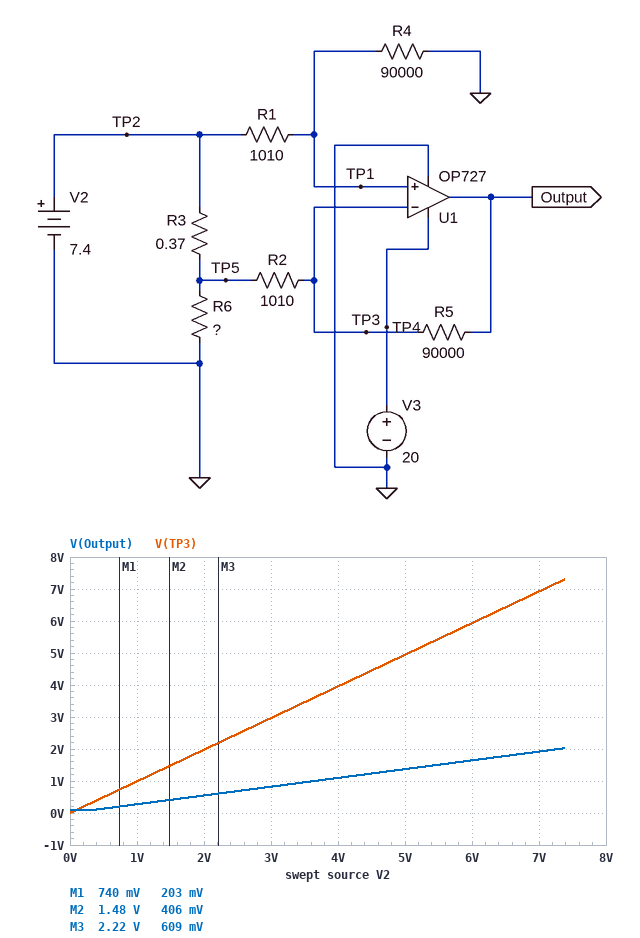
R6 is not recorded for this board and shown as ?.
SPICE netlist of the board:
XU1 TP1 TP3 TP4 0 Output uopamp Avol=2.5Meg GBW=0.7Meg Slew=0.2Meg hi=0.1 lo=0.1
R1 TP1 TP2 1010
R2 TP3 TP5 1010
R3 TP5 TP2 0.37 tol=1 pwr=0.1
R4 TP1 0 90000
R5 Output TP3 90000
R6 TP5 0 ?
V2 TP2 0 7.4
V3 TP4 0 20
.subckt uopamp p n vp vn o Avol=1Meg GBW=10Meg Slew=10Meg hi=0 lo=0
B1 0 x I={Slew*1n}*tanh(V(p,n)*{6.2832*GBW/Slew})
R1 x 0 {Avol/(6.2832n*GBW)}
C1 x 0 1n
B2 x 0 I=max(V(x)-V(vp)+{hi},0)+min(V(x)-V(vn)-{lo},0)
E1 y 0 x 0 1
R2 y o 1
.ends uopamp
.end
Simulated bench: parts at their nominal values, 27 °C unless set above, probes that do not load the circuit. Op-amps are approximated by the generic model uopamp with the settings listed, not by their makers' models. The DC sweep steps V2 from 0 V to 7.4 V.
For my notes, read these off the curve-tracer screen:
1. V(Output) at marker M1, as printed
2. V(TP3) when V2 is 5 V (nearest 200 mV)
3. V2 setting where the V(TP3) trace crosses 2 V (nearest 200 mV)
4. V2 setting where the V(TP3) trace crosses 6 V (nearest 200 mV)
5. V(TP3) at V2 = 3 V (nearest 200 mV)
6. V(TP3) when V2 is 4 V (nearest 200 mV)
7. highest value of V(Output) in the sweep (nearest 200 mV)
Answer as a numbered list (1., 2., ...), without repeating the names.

1. 203 mV
2. 5.0 V
3. 2.0 V
4. 6.0 V
5. 3.0 V
6. 4.0 V
7. 2.0 V
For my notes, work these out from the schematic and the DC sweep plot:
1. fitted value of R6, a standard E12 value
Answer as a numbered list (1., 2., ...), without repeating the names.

1. 120 Ω
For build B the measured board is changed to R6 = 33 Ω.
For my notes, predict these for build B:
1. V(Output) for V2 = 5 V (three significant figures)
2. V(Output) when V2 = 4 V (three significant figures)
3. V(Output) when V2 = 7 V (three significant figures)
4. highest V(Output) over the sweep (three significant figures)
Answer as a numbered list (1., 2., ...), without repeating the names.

1. 4.94 V
2. 3.95 V
3. 6.92 V
4. 7.31 V
